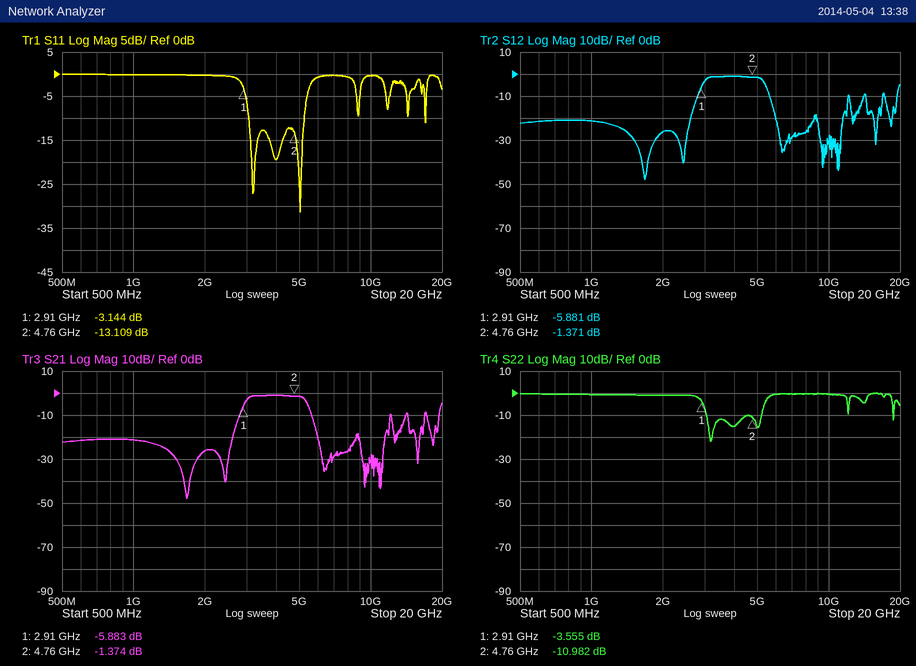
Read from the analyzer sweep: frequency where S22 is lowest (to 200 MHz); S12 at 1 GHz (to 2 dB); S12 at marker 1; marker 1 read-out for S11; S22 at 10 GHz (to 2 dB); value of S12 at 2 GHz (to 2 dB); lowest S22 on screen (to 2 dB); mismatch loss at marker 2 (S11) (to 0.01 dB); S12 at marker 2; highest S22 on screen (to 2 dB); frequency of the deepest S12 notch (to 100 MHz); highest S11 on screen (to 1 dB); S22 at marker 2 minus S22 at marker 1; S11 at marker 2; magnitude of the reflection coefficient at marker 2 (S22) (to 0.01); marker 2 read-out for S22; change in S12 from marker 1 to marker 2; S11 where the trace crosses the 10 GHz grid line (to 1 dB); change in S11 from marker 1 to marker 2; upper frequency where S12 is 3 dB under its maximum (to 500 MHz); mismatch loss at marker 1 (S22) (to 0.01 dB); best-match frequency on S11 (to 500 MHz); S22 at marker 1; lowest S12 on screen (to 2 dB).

3.2 GHz
-22 dB
-5.881 dB
-3.144 dB
0 dB
-26 dB
-22 dB
0.22 dB
-1.371 dB
0 dB
1.7 GHz
0 dB
-7.427 dB
-13.109 dB
0.28
-10.982 dB
4.510 dB
0 dB
-9.965 dB
5.5 GHz
2.53 dB
5.0 GHz
-3.555 dB
-48 dB
